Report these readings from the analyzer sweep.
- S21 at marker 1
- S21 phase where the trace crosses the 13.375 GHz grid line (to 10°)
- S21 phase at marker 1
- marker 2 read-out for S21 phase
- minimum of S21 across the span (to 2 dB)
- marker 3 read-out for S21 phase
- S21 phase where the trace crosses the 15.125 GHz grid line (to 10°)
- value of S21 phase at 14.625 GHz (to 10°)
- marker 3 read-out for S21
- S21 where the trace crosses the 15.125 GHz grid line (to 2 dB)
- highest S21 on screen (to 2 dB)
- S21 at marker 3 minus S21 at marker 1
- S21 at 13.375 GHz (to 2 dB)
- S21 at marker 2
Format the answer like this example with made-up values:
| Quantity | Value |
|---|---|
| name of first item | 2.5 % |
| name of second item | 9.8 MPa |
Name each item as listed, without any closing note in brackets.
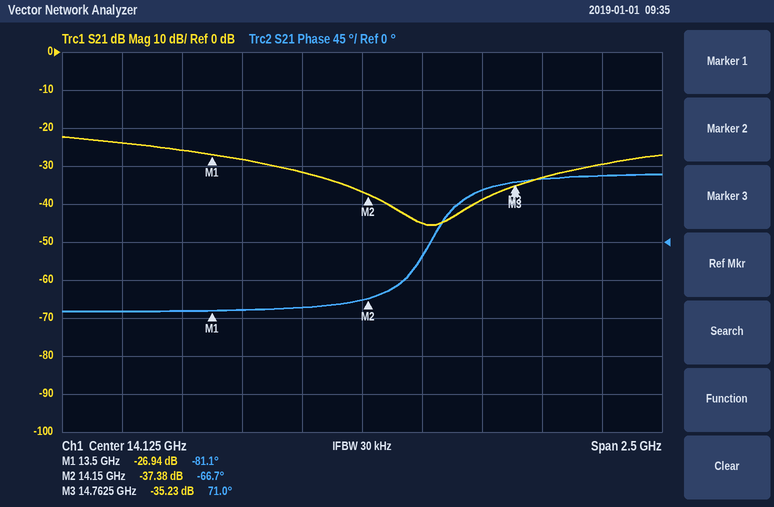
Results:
| Quantity | Value |
|---|---|
| S21 at marker 1 | -26.94 dB |
| S21 phase where the trace crosses the 13.375 GHz grid line | -80° |
| S21 phase at marker 1 | -81.1° |
| marker 2 read-out for S21 phase | -66.7° |
| minimum of S21 across the span | -46 dB |
| marker 3 read-out for S21 phase | 71.0° |
| S21 phase where the trace crosses the 15.125 GHz grid line | 80° |
| value of S21 phase at 14.625 GHz | 60° |
| marker 3 read-out for S21 | -35.23 dB |
| S21 where the trace crosses the 15.125 GHz grid line | -30 dB |
| highest S21 on screen | -22 dB |
| S21 at marker 3 minus S21 at marker 1 | -8.29 dB |
| S21 at 13.375 GHz | -26 dB |
| S21 at marker 2 | -37.38 dB |
